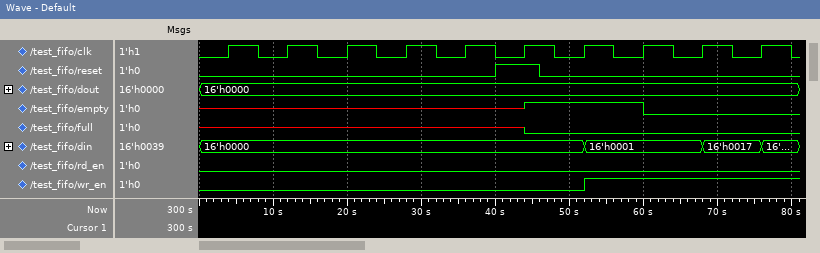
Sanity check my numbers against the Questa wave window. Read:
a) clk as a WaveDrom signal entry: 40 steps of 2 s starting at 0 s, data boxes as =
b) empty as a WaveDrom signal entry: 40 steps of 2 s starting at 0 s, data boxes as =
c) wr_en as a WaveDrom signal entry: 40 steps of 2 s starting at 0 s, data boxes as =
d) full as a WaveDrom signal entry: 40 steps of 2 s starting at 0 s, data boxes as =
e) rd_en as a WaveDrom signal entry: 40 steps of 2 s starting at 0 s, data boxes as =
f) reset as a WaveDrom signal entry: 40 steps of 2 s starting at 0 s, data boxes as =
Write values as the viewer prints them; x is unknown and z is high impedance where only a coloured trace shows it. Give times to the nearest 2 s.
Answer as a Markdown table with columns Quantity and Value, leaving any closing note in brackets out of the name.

| Quantity | Value |
|---|---|
| clk as a WaveDrom signal entry: 40 steps of 2 s starting at 0 s, data boxes as = | {name: 'clk', wave: '0.1.0.1.0.1.0.1.0.1.0.1.0.1.0.1.0.1.0.1.'} |
| empty as a WaveDrom signal entry: 40 steps of 2 s starting at 0 s, data boxes as = | {name: 'empty', wave: 'x.....................1.......0.........'} |
| wr_en as a WaveDrom signal entry: 40 steps of 2 s starting at 0 s, data boxes as = | {name: 'wr_en', wave: '0.........................1.............'} |
| full as a WaveDrom signal entry: 40 steps of 2 s starting at 0 s, data boxes as = | {name: 'full', wave: 'x.....................0.................'} |
| rd_en as a WaveDrom signal entry: 40 steps of 2 s starting at 0 s, data boxes as = | {name: 'rd_en', wave: '0.......................................'} |
| reset as a WaveDrom signal entry: 40 steps of 2 s starting at 0 s, data boxes as = | {name: 'reset', wave: '0...................1..0................'} |
